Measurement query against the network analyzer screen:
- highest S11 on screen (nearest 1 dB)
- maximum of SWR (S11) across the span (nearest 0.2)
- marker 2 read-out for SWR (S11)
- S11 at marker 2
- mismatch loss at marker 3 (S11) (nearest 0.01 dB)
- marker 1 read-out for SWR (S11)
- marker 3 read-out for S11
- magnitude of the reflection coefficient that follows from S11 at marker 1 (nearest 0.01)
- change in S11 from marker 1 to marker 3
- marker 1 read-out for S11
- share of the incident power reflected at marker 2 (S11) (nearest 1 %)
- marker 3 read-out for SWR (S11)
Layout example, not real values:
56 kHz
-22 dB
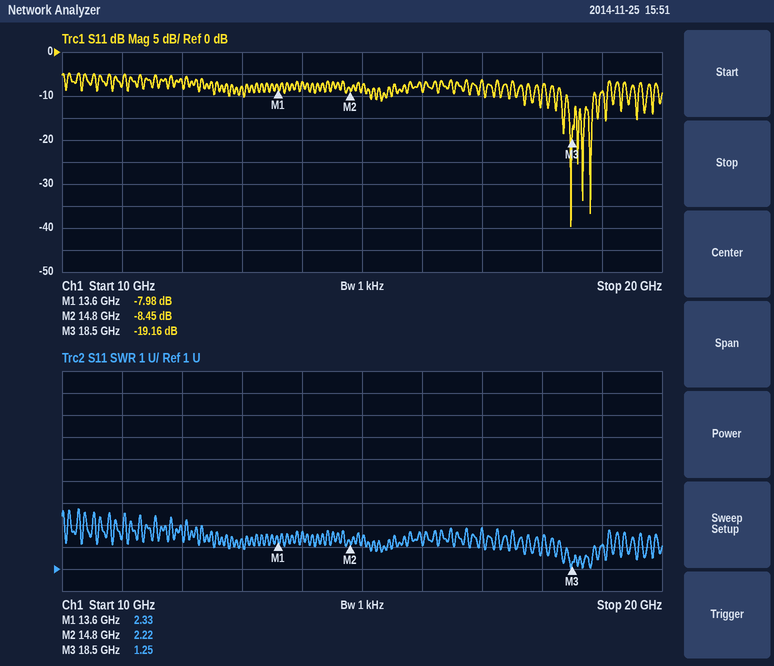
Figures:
-5 dB
3.8
2.22
-8.45 dB
0.05 dB
2.33
-19.16 dB
0.40
-11.18 dB
-7.98 dB
14 %
1.25
